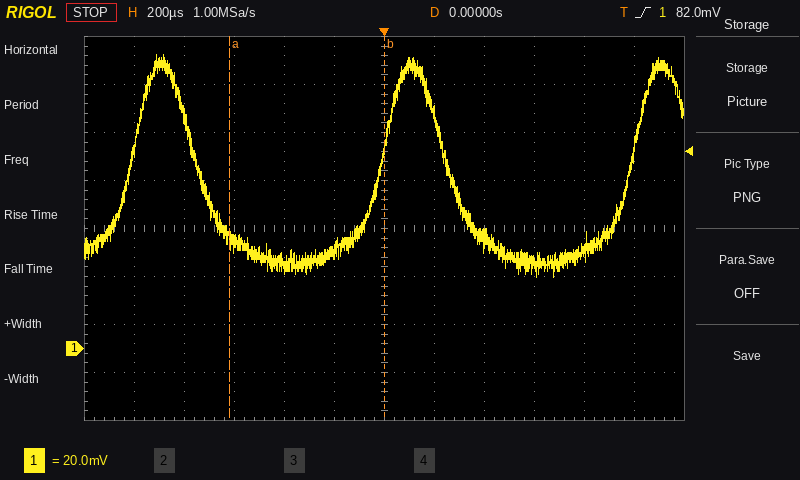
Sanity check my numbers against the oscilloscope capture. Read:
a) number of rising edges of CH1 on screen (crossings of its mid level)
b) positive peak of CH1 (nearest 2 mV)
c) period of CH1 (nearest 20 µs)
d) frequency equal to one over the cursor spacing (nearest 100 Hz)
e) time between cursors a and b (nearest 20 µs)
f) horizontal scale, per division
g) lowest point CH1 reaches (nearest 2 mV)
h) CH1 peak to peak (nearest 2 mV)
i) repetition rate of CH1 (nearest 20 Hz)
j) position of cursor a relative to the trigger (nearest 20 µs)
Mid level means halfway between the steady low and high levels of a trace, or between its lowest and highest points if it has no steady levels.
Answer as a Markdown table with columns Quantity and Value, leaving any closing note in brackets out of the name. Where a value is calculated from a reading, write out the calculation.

| Quantity | Value |
|---|---|
| number of rising edges of CH1 on screen | 3 |
| positive peak of CH1 | 122 mV |
| period of CH1 | 1.00 ms |
| frequency equal to one over the cursor spacing | 1 / 620 µs ≈ 1.6 kHz |
| time between cursors a and b | 620 µs |
| horizontal scale, per division | 200 µs |
| lowest point CH1 reaches | 30 mV |
| CH1 peak to peak | 122 mV − (30 mV) = 92 mV |
| repetition rate of CH1 | 1 / 1.00 ms ≈ 1.00 kHz |
| position of cursor a relative to the trigger | -620 µs |
